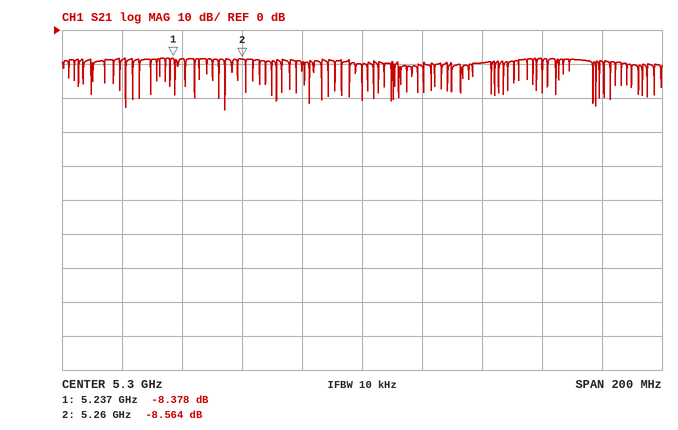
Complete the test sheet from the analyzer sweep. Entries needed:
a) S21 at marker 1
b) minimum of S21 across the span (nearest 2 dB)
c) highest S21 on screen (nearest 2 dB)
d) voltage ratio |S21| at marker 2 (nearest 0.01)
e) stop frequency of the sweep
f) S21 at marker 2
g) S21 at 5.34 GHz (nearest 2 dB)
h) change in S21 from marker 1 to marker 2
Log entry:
-8.378 dB
-24 dB
-8 dB
0.37
5.4 GHz
-8.564 dB
-10 dB
-0.186 dB
